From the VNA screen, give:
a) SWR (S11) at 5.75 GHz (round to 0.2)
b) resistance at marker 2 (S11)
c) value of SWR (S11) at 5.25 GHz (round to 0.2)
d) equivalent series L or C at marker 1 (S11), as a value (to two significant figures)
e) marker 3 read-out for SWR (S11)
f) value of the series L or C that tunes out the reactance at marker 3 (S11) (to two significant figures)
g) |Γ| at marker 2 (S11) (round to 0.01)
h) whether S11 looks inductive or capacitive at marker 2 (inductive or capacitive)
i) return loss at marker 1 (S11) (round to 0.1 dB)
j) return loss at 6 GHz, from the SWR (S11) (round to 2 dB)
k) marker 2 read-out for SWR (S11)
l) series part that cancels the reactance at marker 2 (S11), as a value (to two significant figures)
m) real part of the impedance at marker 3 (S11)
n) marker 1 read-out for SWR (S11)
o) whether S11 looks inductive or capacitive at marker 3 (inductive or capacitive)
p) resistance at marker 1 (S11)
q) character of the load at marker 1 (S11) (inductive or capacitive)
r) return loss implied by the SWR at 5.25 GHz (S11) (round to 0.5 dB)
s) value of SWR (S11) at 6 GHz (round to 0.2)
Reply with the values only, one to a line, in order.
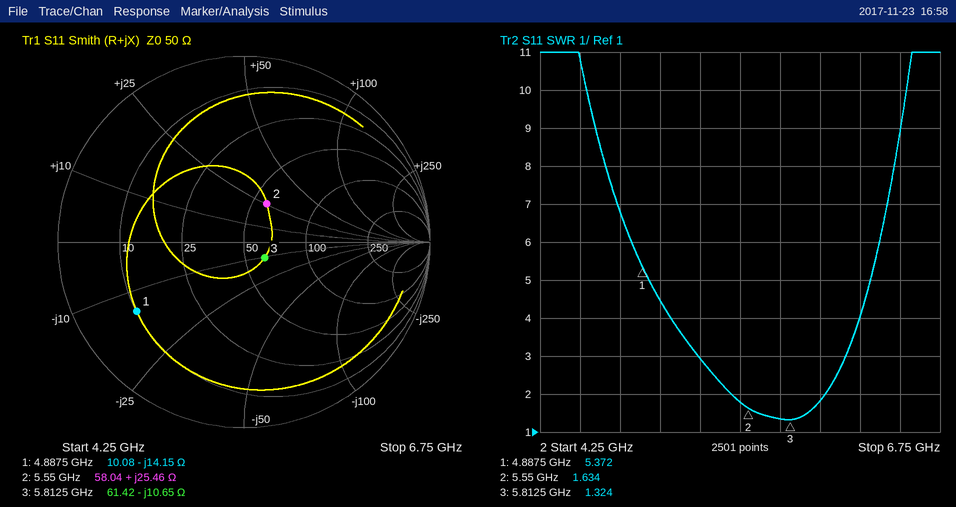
1.4
58.04 Ω
3.0
2.3 pF
1.324
290 pH
0.24
inductive
3.3 dB
10 dB
1.634
1.1 pF
61.42 Ω
5.372
capacitive
10.08 Ω
capacitive
6.0 dB
1.8
